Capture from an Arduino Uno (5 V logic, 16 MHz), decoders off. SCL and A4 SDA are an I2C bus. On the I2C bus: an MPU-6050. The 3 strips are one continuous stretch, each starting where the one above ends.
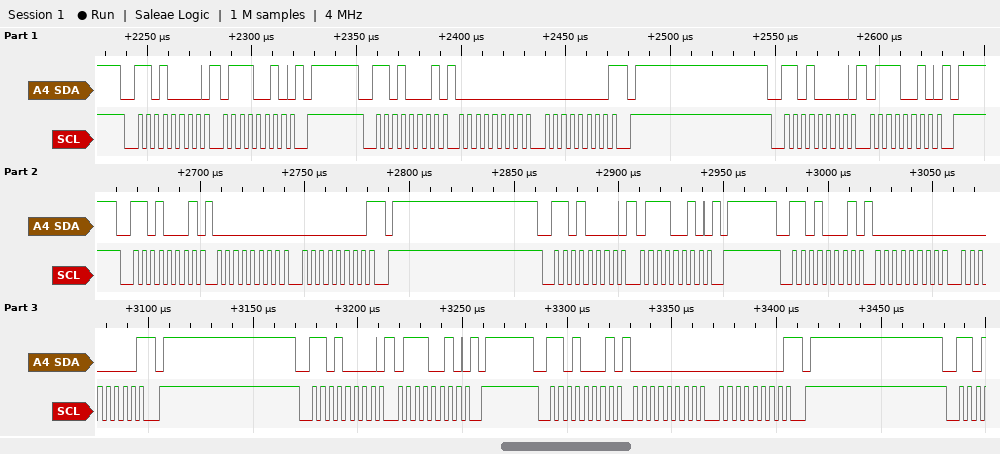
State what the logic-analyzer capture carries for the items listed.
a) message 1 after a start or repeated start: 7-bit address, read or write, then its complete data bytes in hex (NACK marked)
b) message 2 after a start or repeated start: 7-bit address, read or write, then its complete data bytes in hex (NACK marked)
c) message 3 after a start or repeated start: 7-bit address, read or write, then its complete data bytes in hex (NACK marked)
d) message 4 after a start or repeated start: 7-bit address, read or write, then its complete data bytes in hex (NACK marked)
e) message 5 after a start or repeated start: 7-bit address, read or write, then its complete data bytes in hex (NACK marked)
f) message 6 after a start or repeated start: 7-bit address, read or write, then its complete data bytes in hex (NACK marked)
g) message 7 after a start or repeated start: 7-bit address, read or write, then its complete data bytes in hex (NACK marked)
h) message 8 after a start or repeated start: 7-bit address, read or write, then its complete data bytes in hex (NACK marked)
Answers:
0x68 write: 72
0x68 read: 00 00 NACK
0x68 write: 72
0x68 read: 00 00 NACK
0x68 write: 72
0x68 read: 00 00 NACK
0x68 write: 72
0x68 read: 00 00 NACK
